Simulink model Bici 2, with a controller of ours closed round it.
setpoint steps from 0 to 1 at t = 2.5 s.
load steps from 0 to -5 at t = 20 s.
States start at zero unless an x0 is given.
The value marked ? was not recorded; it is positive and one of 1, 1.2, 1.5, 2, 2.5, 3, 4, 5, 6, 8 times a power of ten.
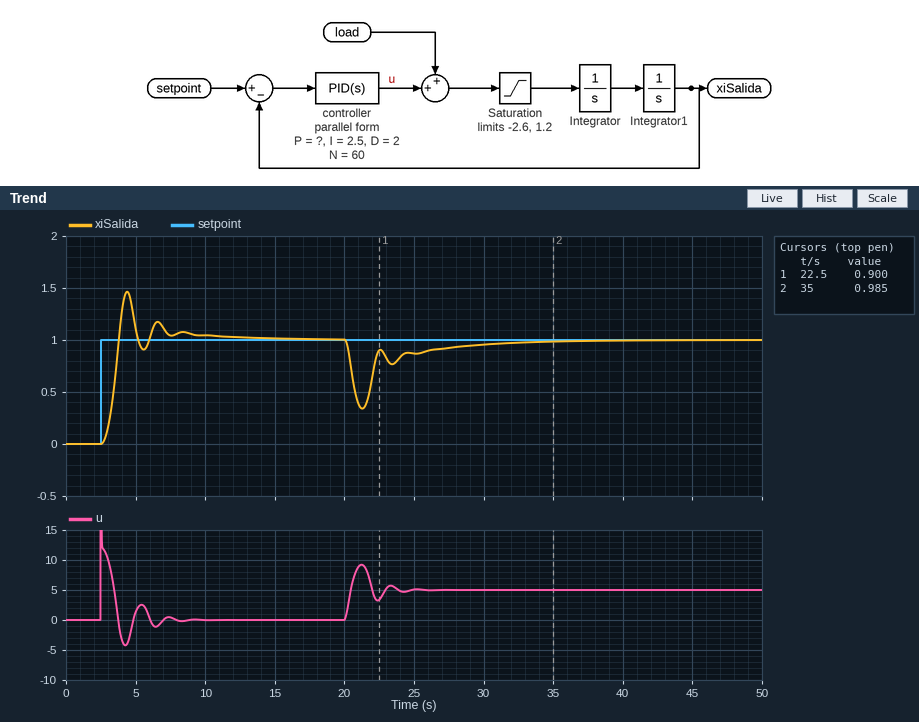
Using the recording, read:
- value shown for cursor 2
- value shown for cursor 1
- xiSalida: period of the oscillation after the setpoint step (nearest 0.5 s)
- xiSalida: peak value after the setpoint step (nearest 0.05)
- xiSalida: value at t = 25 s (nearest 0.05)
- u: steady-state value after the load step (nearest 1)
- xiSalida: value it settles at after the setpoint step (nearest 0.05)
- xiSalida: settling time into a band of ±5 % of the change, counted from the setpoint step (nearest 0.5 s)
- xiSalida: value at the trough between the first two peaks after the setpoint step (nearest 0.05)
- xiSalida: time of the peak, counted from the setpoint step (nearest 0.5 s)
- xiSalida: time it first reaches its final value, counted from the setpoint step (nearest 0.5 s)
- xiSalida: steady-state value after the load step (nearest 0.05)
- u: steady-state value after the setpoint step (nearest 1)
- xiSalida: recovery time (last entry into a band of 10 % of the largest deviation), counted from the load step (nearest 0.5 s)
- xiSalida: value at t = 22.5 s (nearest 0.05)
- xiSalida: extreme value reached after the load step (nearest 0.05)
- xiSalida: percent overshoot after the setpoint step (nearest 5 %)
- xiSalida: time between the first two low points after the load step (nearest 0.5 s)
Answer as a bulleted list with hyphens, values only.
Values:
- 0.985
- 0.900
- 2.0 s
- 1.45
- 0.85
- 5
- 1.00
- 6.5 s
- 0.90
- 2.0 s
- 1.5 s
- 1.00
- 0
- 8.0 s
- 0.90
- 0.35
- 45 %
- 2.0 s
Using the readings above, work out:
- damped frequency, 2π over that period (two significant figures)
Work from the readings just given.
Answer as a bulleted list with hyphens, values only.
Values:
- 3.1 rad/s
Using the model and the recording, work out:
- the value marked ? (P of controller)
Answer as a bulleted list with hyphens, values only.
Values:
- 12
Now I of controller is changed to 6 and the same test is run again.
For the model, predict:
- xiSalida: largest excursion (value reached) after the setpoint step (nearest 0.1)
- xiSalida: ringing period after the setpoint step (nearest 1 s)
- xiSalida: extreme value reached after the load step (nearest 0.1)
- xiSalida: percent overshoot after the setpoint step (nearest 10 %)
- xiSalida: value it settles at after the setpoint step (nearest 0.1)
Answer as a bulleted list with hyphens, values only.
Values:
- 1.8
- 4 s
- 0.4
- 80 %
- 1.0
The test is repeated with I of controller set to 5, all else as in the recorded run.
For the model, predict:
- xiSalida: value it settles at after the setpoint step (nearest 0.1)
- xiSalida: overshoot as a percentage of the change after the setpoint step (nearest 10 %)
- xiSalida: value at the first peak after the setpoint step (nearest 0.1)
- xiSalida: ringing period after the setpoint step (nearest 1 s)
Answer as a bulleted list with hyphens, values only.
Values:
- 1.0
- 70 %
- 1.7
- 3 s
